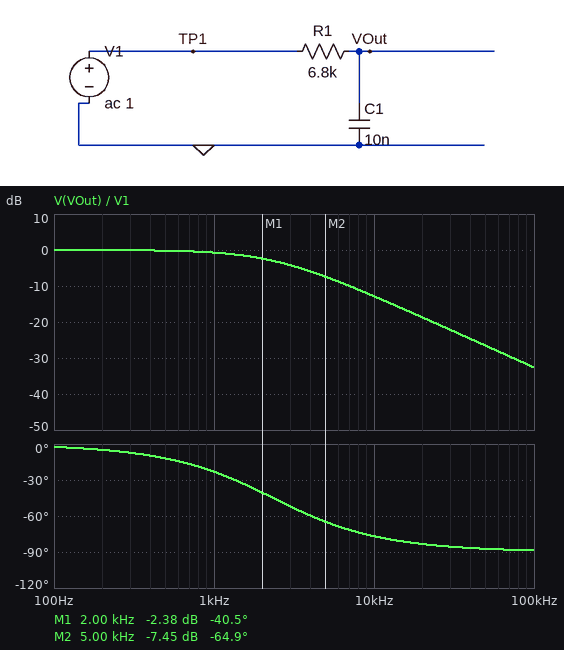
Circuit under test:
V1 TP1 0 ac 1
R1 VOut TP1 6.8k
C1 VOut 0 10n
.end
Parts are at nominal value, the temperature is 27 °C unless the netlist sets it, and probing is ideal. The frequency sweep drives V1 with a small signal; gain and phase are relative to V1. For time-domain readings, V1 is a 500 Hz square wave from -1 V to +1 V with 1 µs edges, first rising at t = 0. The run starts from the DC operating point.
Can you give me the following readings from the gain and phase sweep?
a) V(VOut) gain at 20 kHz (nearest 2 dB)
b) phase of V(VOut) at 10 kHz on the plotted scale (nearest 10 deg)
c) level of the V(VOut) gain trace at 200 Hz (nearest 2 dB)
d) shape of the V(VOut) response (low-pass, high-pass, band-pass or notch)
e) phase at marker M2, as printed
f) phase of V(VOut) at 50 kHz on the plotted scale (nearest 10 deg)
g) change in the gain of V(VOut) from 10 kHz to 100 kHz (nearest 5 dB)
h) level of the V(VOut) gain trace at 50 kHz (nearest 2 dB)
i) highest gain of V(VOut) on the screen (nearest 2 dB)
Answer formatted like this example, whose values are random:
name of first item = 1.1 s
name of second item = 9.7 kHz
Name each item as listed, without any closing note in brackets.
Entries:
V(VOut) gain at 20 kHz = -18 dB
phase of V(VOut) at 10 kHz on the plotted scale = -80 deg
level of the V(VOut) gain trace at 200 Hz = 0 dB
shape of the V(VOut) response = low-pass
phase at marker M2, as printed = -64.9 deg
phase of V(VOut) at 50 kHz on the plotted scale = -90 deg
change in the gain of V(VOut) from 10 kHz to 100 kHz = -20 dB
level of the V(VOut) gain trace at 50 kHz = -26 dB
highest gain of V(VOut) on the screen = 0 dB
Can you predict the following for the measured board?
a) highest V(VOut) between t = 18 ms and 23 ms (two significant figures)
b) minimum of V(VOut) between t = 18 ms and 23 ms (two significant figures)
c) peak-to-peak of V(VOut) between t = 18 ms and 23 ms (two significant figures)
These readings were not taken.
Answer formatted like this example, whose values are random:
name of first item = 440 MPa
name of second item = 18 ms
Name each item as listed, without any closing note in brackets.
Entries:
highest V(VOut) between t = 18 ms and 23 ms = 1.0 V
minimum of V(VOut) between t = 18 ms and 23 ms = -1.0 V
peak-to-peak of V(VOut) between t = 18 ms and 23 ms = 2.0 V
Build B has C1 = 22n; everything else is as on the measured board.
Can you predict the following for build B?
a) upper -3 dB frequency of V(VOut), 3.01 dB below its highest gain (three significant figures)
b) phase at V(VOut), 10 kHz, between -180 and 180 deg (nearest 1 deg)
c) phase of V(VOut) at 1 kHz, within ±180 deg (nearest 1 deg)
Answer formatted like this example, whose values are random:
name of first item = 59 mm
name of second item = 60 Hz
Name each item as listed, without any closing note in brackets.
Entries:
upper -3 dB frequency of V(VOut), 3.01 dB below its highest gain = 1.06 kHz
phase at V(VOut), 10 kHz, between -180 and 180 deg = -84 deg
phase of V(VOut) at 1 kHz, within ±180 deg = -43 deg
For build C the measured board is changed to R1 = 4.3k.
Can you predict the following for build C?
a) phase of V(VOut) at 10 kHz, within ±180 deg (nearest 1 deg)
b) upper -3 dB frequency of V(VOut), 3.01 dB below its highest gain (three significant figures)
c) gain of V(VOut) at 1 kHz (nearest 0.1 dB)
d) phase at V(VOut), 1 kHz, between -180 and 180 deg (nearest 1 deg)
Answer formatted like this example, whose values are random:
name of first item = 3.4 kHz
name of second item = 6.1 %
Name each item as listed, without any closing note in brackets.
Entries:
phase of V(VOut) at 10 kHz, within ±180 deg = -70 deg
upper -3 dB frequency of V(VOut), 3.01 dB below its highest gain = 3.70 kHz
gain of V(VOut) at 1 kHz = -0.3 dB
phase at V(VOut), 1 kHz, between -180 and 180 deg = -15 deg
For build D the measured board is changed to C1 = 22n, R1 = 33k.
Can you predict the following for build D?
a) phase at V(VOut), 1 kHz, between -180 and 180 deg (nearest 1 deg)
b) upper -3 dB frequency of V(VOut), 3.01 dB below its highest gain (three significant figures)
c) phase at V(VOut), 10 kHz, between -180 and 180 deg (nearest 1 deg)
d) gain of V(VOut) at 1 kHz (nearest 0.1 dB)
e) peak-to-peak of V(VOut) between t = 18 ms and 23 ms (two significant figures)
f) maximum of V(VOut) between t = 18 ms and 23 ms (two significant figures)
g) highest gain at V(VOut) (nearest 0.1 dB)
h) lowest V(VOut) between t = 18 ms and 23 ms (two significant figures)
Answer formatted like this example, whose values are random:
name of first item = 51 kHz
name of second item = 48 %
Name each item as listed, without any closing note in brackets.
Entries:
phase at V(VOut), 1 kHz, between -180 and 180 deg = -78 deg
upper -3 dB frequency of V(VOut), 3.01 dB below its highest gain = 219 Hz
phase at V(VOut), 10 kHz, between -180 and 180 deg = -89 deg
gain of V(VOut) at 1 kHz = -13.4 dB
peak-to-peak of V(VOut) between t = 18 ms and 23 ms = 1.2 V
maximum of V(VOut) between t = 18 ms and 23 ms = 600 mV
highest gain at V(VOut) = 0 dB
lowest V(VOut) between t = 18 ms and 23 ms = -600 mV
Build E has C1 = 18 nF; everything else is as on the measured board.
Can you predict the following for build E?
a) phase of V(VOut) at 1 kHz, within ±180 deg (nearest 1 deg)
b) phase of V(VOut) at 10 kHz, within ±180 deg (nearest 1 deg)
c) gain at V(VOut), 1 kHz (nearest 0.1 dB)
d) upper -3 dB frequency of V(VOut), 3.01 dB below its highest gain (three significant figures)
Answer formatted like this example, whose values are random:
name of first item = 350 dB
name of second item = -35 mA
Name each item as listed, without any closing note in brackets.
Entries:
phase of V(VOut) at 1 kHz, within ±180 deg = -38 deg
phase of V(VOut) at 10 kHz, within ±180 deg = -83 deg
gain at V(VOut), 1 kHz = -2.0 dB
upper -3 dB frequency of V(VOut), 3.01 dB below its highest gain = 1.30 kHz
